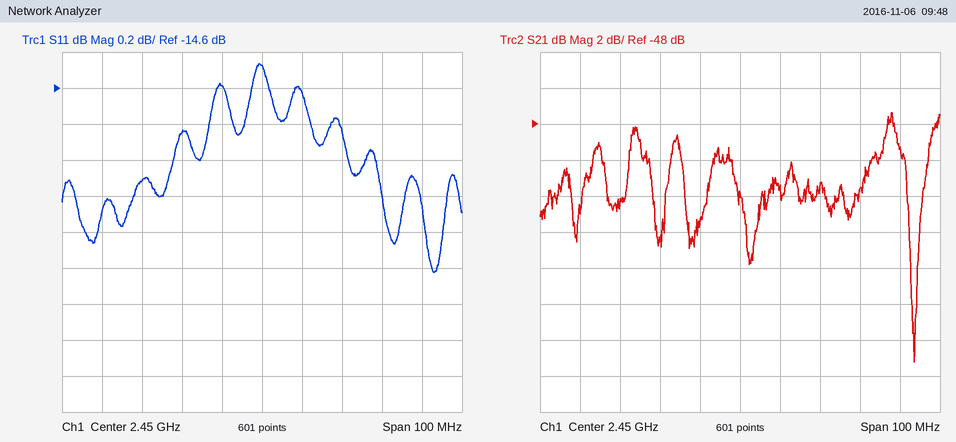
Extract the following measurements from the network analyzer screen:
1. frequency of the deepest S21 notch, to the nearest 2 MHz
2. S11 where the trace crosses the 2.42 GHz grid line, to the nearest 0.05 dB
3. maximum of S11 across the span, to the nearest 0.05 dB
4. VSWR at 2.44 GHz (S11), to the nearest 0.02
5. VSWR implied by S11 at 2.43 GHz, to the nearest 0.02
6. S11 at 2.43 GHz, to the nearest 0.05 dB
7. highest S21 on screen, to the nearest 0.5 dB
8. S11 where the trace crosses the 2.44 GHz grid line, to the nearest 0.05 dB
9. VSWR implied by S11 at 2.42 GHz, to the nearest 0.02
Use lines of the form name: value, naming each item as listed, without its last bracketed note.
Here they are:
frequency of the deepest S21 notch, to the nearest 2 MHz: 2.494 GHz
S11 where the trace crosses the 2.42 GHz grid line, to the nearest 0.05 dB: -15.10 dB
maximum of S11 across the span, to the nearest 0.05 dB: -14.45 dB
VSWR at 2.44 GHz (S11), to the nearest 0.02: 1.46
VSWR implied by S11 at 2.43 GHz, to the nearest 0.02: 1.44
S11 at 2.43 GHz, to the nearest 0.05 dB: -14.85 dB
highest S21 on screen, to the nearest 0.5 dB: -47.5 dB
S11 where the trace crosses the 2.44 GHz grid line, to the nearest 0.05 dB: -14.60 dB
VSWR implied by S11 at 2.42 GHz, to the nearest 0.02: 1.42
